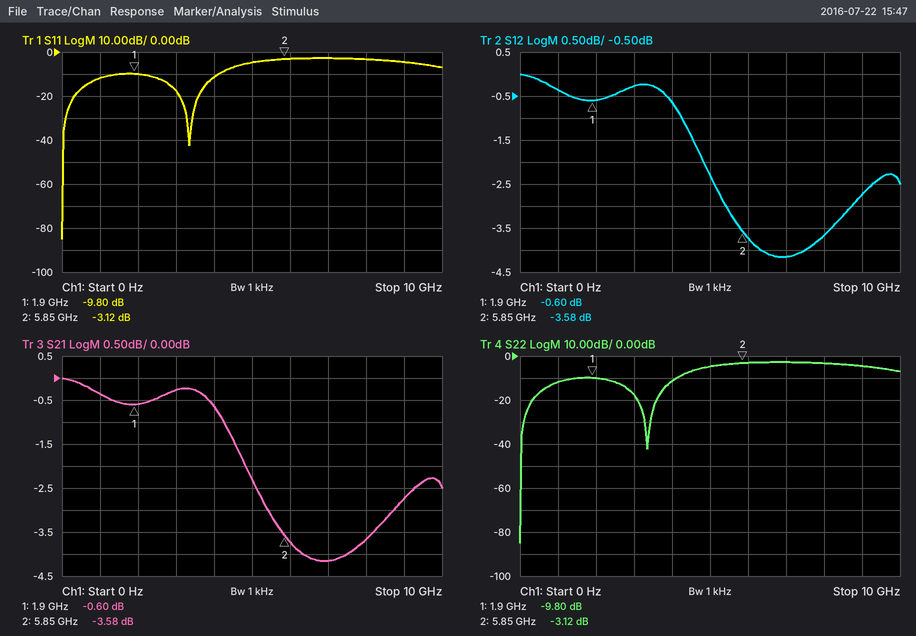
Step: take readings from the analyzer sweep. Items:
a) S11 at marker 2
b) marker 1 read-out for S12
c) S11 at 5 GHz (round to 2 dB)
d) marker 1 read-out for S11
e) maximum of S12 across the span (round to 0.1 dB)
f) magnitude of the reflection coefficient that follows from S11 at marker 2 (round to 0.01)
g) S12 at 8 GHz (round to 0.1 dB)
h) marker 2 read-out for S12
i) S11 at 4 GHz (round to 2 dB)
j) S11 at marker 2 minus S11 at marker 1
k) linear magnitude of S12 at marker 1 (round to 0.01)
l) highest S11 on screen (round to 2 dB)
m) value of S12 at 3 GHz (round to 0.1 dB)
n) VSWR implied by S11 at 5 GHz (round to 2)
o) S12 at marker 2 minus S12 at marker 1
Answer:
-3.12 dB
-0.60 dB
-4 dB
-9.80 dB
0.0 dB
0.70
-3.7 dB
-3.58 dB
-12 dB
6.68 dB
0.93
-2 dB
-0.3 dB
4
-2.98 dB
